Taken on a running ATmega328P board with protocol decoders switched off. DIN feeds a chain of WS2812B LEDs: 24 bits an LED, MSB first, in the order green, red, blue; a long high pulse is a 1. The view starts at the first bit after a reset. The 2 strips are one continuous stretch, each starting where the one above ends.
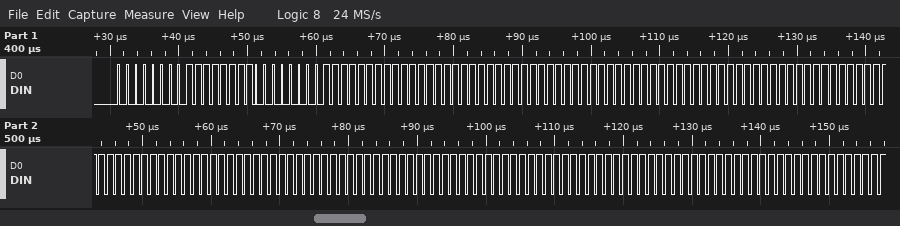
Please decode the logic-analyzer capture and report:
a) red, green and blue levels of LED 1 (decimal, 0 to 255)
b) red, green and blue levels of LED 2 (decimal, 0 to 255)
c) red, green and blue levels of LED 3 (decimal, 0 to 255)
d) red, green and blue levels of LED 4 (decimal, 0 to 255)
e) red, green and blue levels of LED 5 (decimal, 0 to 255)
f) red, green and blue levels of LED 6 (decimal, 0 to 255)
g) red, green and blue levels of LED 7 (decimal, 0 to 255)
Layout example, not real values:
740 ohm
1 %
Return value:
255, 0, 0
255, 255, 255
255, 255, 255
255, 255, 255
255, 255, 255
255, 255, 255
255, 255, 255
